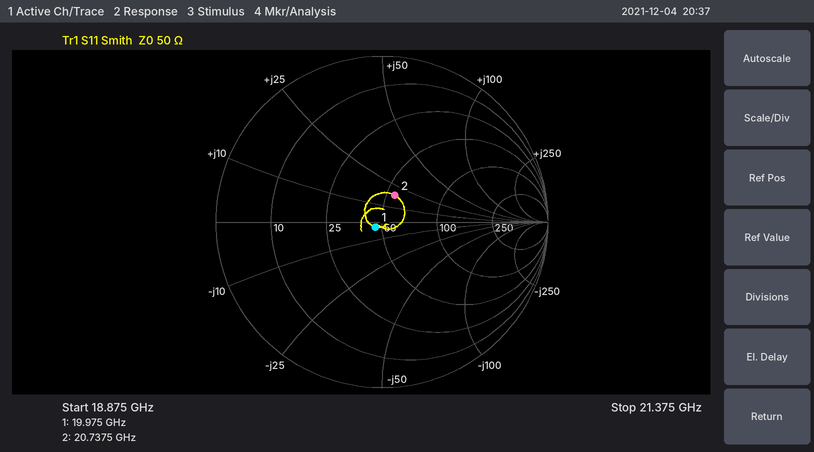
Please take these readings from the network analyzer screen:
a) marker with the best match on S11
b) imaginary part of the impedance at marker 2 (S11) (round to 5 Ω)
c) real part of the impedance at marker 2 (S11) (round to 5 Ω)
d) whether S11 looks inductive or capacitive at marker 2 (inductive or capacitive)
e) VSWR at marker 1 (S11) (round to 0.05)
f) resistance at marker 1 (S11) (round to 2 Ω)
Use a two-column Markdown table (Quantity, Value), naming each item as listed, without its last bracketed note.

| Quantity | Value |
|---|---|
| marker with the best match on S11 | marker 1 |
| imaginary part of the impedance at marker 2 (S11) | +20 Ω |
| real part of the impedance at marker 2 (S11) | 55 Ω |
| whether S11 looks inductive or capacitive at marker 2 | inductive |
| VSWR at marker 1 (S11) | 1.10 |
| resistance at marker 1 (S11) | 46 Ω |
